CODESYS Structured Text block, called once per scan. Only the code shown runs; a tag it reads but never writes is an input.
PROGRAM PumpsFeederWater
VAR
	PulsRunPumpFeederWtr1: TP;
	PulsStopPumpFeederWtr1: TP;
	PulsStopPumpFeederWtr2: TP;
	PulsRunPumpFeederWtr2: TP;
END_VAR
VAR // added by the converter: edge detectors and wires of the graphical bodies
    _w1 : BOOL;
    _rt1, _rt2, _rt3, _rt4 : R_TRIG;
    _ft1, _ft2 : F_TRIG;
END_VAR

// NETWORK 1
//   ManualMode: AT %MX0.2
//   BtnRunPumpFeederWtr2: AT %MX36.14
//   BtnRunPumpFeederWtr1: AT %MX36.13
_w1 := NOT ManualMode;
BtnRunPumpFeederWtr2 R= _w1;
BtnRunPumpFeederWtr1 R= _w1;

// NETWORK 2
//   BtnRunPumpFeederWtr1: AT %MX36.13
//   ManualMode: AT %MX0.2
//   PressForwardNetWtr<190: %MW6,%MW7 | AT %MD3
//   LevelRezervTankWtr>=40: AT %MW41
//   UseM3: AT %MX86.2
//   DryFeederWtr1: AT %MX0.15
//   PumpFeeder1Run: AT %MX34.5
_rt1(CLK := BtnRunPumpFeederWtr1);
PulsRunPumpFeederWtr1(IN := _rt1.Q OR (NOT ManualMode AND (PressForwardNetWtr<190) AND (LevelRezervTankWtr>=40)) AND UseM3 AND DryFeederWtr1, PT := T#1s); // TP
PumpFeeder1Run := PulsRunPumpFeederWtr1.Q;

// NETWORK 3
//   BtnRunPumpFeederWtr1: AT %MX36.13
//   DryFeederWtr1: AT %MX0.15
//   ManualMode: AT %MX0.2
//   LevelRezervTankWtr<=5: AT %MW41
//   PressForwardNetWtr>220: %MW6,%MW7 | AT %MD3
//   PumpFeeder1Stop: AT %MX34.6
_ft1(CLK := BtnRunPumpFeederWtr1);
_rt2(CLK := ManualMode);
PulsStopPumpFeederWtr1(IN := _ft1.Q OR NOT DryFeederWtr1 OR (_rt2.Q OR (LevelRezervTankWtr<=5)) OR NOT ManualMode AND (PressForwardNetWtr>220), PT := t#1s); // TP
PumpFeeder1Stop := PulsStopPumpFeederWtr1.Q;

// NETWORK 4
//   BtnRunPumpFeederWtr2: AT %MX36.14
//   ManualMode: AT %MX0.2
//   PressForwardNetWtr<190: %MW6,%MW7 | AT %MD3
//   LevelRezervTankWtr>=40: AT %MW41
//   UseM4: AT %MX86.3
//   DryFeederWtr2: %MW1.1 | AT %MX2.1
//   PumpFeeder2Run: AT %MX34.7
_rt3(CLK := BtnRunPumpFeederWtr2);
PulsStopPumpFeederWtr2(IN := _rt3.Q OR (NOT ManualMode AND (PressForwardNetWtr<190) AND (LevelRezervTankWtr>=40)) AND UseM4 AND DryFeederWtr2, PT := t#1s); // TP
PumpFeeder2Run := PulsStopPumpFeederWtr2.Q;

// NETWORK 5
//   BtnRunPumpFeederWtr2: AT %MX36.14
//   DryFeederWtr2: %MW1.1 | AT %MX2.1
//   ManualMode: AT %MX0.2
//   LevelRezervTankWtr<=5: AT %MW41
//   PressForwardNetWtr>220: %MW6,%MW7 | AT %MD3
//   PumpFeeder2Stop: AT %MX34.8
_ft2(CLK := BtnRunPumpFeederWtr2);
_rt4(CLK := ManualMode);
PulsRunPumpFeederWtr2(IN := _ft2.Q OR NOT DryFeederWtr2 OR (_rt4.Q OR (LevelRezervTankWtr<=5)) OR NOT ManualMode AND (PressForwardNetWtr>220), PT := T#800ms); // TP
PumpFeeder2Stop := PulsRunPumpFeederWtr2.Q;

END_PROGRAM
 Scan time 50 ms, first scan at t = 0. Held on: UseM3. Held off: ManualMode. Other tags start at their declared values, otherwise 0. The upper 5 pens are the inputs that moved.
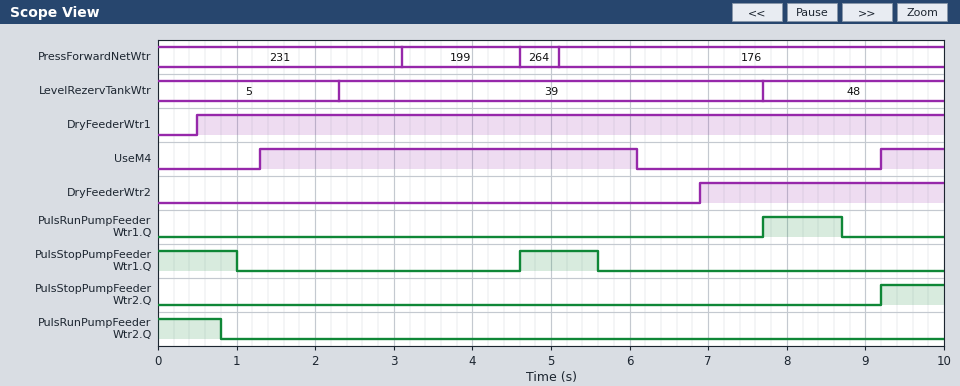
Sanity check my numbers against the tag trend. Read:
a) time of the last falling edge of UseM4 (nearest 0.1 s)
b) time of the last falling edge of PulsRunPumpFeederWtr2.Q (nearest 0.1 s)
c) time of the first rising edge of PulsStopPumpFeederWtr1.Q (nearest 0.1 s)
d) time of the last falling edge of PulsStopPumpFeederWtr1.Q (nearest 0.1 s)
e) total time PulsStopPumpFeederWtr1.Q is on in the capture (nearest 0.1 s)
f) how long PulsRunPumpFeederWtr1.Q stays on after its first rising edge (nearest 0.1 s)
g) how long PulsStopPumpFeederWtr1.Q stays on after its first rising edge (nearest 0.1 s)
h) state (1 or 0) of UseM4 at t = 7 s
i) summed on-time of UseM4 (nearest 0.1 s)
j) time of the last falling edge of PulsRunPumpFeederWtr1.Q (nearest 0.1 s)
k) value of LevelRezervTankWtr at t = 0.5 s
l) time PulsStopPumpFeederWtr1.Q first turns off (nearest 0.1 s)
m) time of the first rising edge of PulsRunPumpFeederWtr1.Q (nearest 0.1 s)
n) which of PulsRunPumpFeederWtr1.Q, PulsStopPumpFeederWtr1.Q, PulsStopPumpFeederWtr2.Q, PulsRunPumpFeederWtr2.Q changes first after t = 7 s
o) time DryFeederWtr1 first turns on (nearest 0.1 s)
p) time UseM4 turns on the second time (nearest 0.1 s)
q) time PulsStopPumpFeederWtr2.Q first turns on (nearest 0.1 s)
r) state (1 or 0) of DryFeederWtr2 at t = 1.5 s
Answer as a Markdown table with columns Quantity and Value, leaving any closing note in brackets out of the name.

| Quantity | Value |
|---|---|
| time of the last falling edge of UseM4 | 6.1 s |
| time of the last falling edge of PulsRunPumpFeederWtr2.Q | 0.8 s |
| time of the first rising edge of PulsStopPumpFeederWtr1.Q | 4.6 s |
| time of the last falling edge of PulsStopPumpFeederWtr1.Q | 5.6 s |
| total time PulsStopPumpFeederWtr1.Q is on in the capture | 2.0 s |
| how long PulsRunPumpFeederWtr1.Q stays on after its first rising edge | 1.0 s |
| how long PulsStopPumpFeederWtr1.Q stays on after its first rising edge | 1.0 s |
| state (1 or 0) of UseM4 at t = 7 s | 0 |
| summed on-time of UseM4 | 5.6 s |
| time of the last falling edge of PulsRunPumpFeederWtr1.Q | 8.7 s |
| value of LevelRezervTankWtr at t = 0.5 s | 5 |
| time PulsStopPumpFeederWtr1.Q first turns off | 1.0 s |
| time of the first rising edge of PulsRunPumpFeederWtr1.Q | 7.7 s |
| which of PulsRunPumpFeederWtr1.Q, PulsStopPumpFeederWtr1.Q, PulsStopPumpFeederWtr2.Q, PulsRunPumpFeederWtr2.Q changes first after t = 7 s | PulsRunPumpFeederWtr1.Q |
| time DryFeederWtr1 first turns on | 0.5 s |
| time UseM4 turns on the second time | 9.2 s |
| time PulsStopPumpFeederWtr2.Q first turns on | 9.2 s |
| state (1 or 0) of DryFeederWtr2 at t = 1.5 s | 0 |
